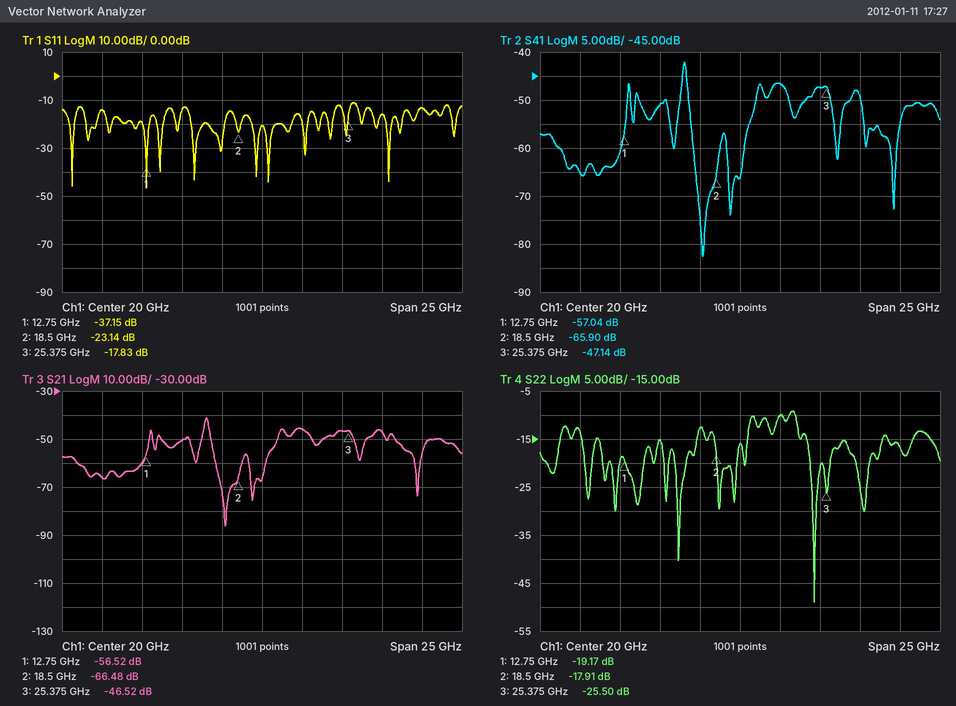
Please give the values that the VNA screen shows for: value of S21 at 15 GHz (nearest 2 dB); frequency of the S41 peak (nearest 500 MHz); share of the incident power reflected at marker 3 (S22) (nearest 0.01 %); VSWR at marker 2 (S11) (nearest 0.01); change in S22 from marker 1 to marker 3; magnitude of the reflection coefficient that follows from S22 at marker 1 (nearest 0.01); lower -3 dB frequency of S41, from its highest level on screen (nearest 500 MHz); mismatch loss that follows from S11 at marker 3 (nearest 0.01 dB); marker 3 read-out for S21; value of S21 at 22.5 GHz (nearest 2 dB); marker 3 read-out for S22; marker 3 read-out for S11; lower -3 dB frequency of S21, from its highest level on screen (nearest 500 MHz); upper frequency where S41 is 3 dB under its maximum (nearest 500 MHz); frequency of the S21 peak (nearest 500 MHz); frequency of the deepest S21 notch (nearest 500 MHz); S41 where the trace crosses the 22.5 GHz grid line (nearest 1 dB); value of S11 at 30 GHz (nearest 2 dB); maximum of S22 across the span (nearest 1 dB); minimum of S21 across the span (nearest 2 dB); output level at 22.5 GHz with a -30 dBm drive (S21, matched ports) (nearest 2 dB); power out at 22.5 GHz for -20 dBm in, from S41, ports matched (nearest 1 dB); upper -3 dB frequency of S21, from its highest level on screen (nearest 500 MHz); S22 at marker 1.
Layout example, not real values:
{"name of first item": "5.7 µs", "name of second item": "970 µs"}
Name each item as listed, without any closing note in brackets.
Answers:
{"value of S21 at 15 GHz": "-50 dB", "frequency of the S41 peak": "16.5 GHz", "share of the incident power reflected at marker 3 (S22)": "0.28 %", "VSWR at marker 2 (S11)": "1.15", "change in S22 from marker 1 to marker 3": "-6.33 dB", "magnitude of the reflection coefficient that follows from S22 at marker 1": "0.11", "lower -3 dB frequency of S41, from its highest level on screen": "16.5 GHz", "mismatch loss that follows from S11 at marker 3": "0.07 dB", "marker 3 read-out for S21": "-46.52 dB", "value of S21 at 22.5 GHz": "-46 dB", "marker 3 read-out for S22": "-25.50 dB", "marker 3 read-out for S11": "-17.83 dB", "lower -3 dB frequency of S21, from its highest level on screen": "16.5 GHz", "upper frequency where S41 is 3 dB under its maximum": "16.5 GHz", "frequency of the S21 peak": "16.5 GHz", "frequency of the deepest S21 notch": "17.5 GHz", "S41 where the trace crosses the 22.5 GHz grid line": "-47 dB", "value of S11 at 30 GHz": "-14 dB", "maximum of S22 across the span": "-9 dB", "minimum of S21 across the span": "-86 dB", "output level at 22.5 GHz with a -30 dBm drive (S21, matched ports)": "-76 dBm", "power out at 22.5 GHz for -20 dBm in, from S41, ports matched": "-67 dBm", "upper -3 dB frequency of S21, from its highest level on screen": "16.5 GHz", "S22 at marker 1": "-19.17 dB"}
